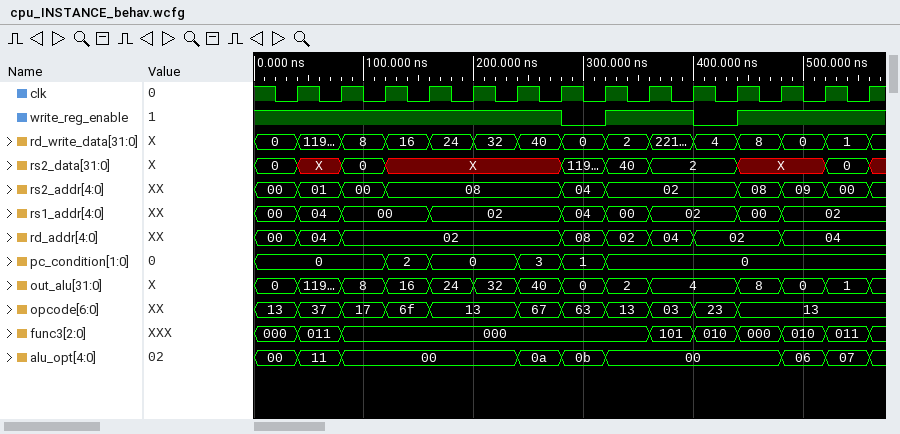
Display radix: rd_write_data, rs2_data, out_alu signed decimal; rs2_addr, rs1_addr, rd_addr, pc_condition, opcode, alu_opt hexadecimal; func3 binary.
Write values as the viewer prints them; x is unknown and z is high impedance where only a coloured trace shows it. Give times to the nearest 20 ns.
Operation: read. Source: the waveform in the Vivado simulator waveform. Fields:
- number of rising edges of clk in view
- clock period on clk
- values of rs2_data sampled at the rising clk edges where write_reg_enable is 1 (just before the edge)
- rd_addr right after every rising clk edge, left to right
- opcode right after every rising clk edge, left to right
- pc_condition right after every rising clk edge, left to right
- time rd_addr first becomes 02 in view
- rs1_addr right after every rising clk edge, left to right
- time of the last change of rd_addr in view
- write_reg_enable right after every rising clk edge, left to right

14
40 ns
0, X, 0, X, X, X, X, 40, 2, X, X, 0
04, 02, 02, 02, 02, 02, 08, 02, 04, 02, 02, 04, 04, 04
37, 17, 6f, 13, 13, 67, 63, 13, 03, 23, 13, 13, 13, 13
0, 0, 2, 0, 0, 3, 1, 0, 0, 0, 0, 0, 0, 0
80 ns
04, 00, 00, 02, 02, 02, 04, 00, 02, 02, 00, 02, 02, 02
480 ns
1 1 1 1 1 1 0 1 1 0 1 1 1 1
